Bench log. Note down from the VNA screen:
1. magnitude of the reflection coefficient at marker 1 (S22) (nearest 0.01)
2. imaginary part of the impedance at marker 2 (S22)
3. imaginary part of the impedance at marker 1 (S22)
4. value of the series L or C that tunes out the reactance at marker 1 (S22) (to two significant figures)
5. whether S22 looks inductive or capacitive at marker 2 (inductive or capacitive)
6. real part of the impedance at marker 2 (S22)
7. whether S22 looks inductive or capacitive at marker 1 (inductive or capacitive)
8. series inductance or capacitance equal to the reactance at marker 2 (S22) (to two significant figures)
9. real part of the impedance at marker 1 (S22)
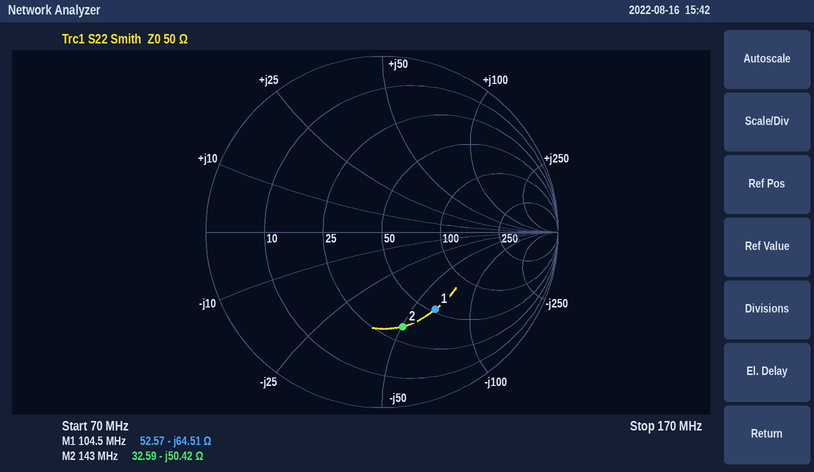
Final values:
0.53
-50.42 Ω
-64.51 Ω
98 nH
capacitive
32.59 Ω
capacitive
22 pF
52.57 Ω
